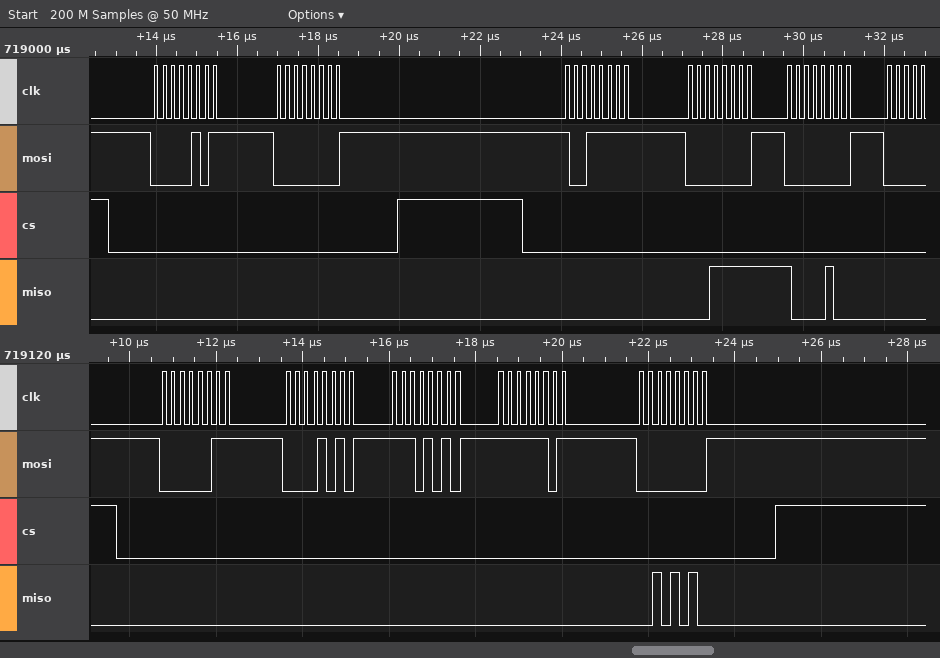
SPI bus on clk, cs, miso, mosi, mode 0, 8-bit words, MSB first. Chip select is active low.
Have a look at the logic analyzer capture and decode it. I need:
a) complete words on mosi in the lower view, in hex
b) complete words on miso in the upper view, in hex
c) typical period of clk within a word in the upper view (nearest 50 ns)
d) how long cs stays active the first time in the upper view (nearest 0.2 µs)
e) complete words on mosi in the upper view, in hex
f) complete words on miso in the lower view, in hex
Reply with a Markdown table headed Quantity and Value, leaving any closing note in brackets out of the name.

| Quantity | Value |
|---|---|
| complete words on mosi in the lower view, in hex | 03, 0A, EA, FD, 00 |
| complete words on miso in the upper view, in hex | 00, 00, 00, 1F, 84 |
| typical period of clk within a word in the upper view | 200 ns |
| how long cs stays active the first time in the upper view | 7.2 µs |
| complete words on mosi in the upper view, in hex | 05, 00, 9F, 00, 00 |
| complete words on miso in the lower view, in hex | 00, 00, 00, 00, 2A |
